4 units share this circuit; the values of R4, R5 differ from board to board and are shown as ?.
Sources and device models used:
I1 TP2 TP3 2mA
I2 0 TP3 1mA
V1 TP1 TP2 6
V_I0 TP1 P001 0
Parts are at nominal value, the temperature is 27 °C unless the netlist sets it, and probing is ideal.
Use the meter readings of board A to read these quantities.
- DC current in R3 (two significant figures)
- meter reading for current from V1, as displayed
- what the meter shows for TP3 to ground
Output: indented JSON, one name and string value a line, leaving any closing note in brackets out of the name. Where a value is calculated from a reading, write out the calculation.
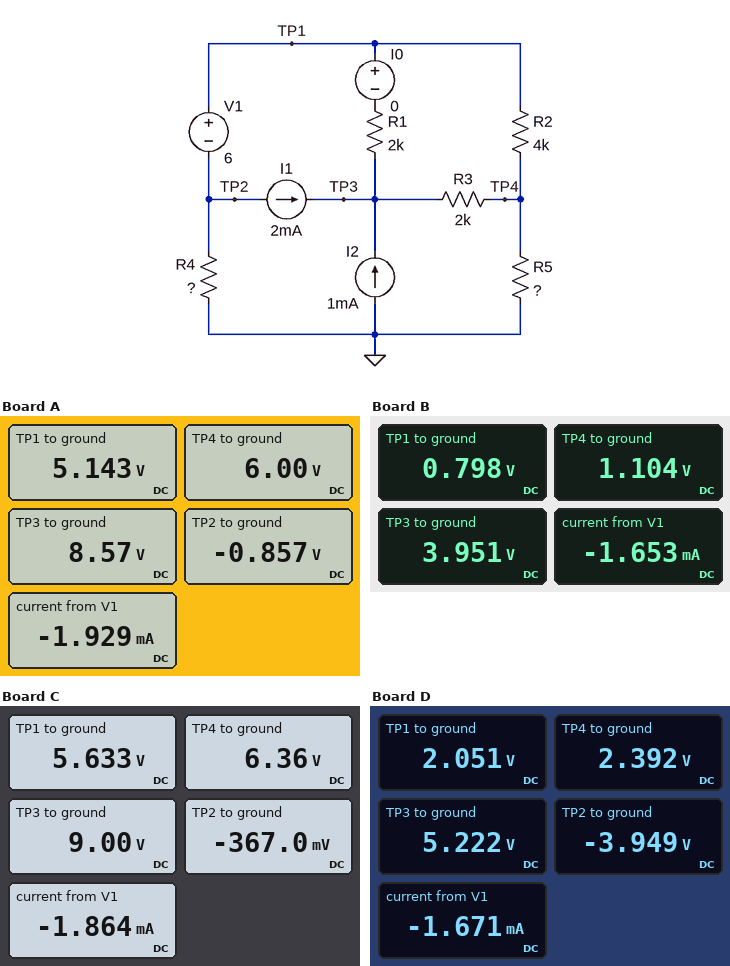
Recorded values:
{
  "DC current in R3": "(8.57 V - 6 V) / 2 kΩ = 1.3 mA",
  "meter reading for current from V1, as displayed": "-1.929 mA",
  "what the meter shows for TP3 to ground": "8.57 V"
}
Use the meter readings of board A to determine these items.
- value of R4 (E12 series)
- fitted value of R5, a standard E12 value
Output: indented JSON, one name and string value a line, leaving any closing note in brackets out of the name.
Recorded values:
{
  "value of R4": "12 kΩ",
  "fitted value of R5, a standard E12 value": "5.6 kΩ"
}
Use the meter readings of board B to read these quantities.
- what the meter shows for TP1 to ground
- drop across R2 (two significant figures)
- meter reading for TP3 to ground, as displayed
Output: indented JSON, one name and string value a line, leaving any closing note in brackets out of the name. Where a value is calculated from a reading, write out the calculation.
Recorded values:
{
  "what the meter shows for TP1 to ground": "0.798 V",
  "drop across R2": "1.104 V - 798 mV = 310 mV",
  "meter reading for TP3 to ground, as displayed": "3.951 V"
}
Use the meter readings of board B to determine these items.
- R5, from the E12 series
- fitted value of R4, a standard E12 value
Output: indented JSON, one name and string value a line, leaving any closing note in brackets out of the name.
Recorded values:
{
  "R5, from the E12 series": "820 Ω",
  "fitted value of R4, a standard E12 value": "15 kΩ"
}
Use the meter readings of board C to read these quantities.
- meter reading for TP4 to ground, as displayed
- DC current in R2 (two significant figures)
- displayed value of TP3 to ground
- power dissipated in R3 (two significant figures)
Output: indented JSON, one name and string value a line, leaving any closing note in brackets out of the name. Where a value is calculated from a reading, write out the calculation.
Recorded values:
{
  "meter reading for TP4 to ground, as displayed": "6.36 V",
  "DC current in R2": "(6.36 V - 5.633 V) / 4 kΩ = 180 µA",
  "displayed value of TP3 to ground": "9.00 V",
  "power dissipated in R3": "(9 V - 6.36 V)^2 / 2 kΩ = 3.5 mW"
}
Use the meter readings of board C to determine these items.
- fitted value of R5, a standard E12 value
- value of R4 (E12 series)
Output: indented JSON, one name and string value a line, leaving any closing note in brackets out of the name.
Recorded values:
{
  "fitted value of R5, a standard E12 value": "5.6 kΩ",
  "value of R4": "2.7 kΩ"
}
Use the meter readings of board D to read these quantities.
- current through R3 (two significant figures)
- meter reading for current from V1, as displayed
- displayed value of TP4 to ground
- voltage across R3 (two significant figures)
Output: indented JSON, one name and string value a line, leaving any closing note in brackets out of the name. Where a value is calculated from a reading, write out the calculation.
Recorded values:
{
  "current through R3": "(5.222 V - 2.392 V) / 2 kΩ = 1.4 mA",
  "meter reading for current from V1, as displayed": "-1.671 mA",
  "displayed value of TP4 to ground": "2.392 V",
  "voltage across R3": "5.222 V - 2.392 V = 2.8 V"
}
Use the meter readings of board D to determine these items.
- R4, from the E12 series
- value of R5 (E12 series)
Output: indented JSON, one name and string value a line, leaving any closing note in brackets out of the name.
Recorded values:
{
  "R4, from the E12 series": "12 kΩ",
  "value of R5": "1.8 kΩ"
}
